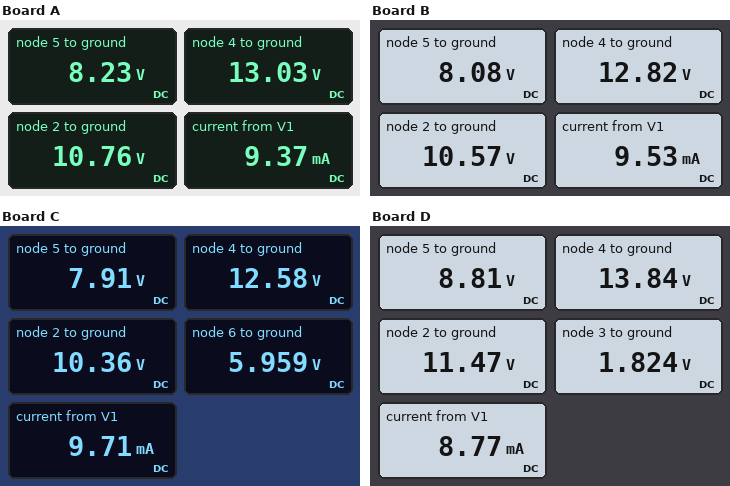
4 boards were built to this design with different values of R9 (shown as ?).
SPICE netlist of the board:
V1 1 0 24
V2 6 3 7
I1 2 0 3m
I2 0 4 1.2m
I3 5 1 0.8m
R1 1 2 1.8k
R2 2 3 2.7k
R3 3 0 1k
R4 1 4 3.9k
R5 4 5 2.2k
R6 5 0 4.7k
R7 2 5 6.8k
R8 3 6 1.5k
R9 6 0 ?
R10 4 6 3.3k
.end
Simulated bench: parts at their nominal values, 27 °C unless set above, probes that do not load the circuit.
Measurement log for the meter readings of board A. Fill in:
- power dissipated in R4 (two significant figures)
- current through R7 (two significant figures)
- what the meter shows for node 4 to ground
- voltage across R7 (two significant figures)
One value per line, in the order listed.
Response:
31 mW
370 µA
13.03 V
2.5 V
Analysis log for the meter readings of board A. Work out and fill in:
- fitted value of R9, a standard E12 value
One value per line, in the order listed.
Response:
1.2 kΩ
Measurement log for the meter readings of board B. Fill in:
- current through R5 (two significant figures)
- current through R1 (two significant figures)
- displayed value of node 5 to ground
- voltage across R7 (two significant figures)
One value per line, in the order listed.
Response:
2.2 mA
7.5 mA
8.08 V
2.5 V
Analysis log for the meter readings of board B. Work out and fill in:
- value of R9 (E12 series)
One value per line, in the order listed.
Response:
1 kΩ
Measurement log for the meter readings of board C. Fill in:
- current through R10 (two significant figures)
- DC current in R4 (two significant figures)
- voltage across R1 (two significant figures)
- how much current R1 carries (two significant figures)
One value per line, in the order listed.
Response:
2.0 mA
2.9 mA
14 V
7.6 mA
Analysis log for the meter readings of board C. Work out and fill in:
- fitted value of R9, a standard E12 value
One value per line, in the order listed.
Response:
820 Ω
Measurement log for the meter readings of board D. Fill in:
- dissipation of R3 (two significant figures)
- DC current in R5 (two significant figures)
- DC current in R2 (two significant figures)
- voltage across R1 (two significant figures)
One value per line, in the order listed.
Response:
3.3 mW
2.3 mA
3.6 mA
13 V
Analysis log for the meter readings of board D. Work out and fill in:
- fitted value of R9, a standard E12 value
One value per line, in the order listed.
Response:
2.7 kΩ
